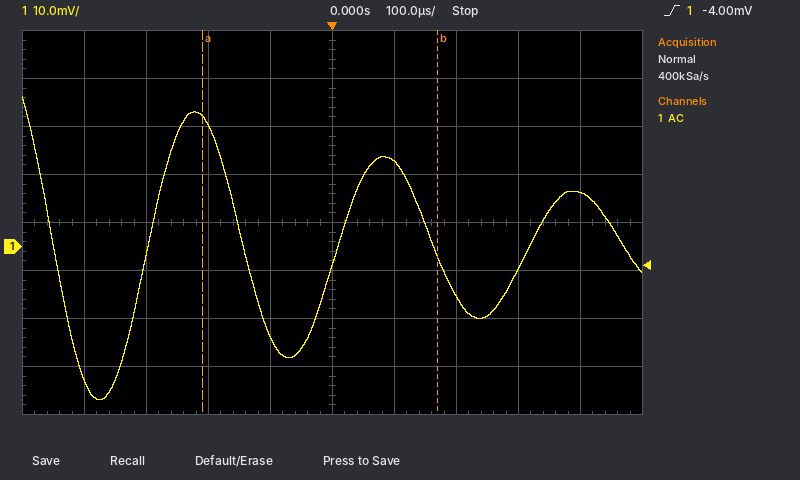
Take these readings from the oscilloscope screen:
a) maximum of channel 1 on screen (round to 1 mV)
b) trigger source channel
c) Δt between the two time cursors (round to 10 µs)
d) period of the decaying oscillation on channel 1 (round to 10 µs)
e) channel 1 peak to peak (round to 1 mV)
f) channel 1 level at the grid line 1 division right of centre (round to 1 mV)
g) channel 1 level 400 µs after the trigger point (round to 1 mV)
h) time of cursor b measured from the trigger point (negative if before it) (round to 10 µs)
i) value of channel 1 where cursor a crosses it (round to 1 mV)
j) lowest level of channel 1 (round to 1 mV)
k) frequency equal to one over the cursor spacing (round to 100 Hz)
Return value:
31 mV
channel 1
380 µs
300 µs
63 mV
18 mV
11 mV
+170 µs
27 mV
-32 mV
2.6 kHz
